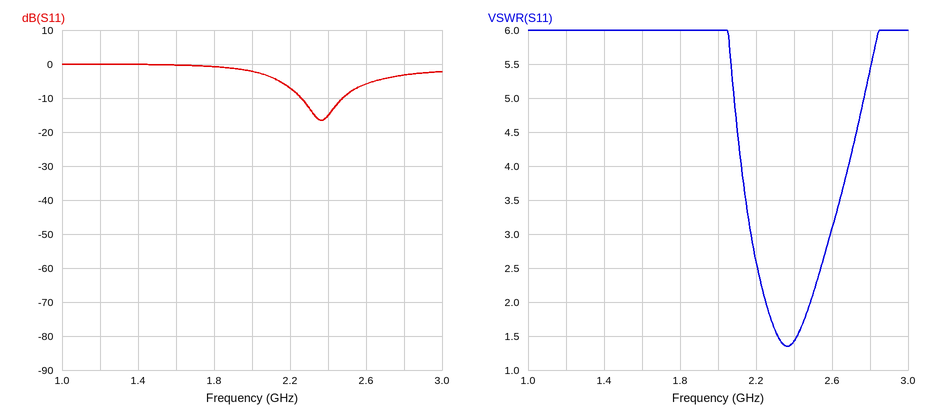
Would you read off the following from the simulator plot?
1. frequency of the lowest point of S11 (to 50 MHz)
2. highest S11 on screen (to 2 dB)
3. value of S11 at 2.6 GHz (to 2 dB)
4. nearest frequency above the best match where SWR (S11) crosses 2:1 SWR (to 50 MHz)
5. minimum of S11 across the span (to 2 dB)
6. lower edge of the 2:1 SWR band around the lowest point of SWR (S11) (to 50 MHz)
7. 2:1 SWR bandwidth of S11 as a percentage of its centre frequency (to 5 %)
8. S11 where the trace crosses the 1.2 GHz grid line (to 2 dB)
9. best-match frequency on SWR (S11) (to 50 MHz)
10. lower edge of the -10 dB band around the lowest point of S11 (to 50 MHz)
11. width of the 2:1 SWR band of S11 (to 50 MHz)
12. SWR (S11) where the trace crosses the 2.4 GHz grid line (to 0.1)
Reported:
2.35 GHz
0 dB
-6 dB
2.50 GHz
-16 dB
2.25 GHz
10 %
0 dB
2.35 GHz
2.25 GHz
250 MHz
1.4
